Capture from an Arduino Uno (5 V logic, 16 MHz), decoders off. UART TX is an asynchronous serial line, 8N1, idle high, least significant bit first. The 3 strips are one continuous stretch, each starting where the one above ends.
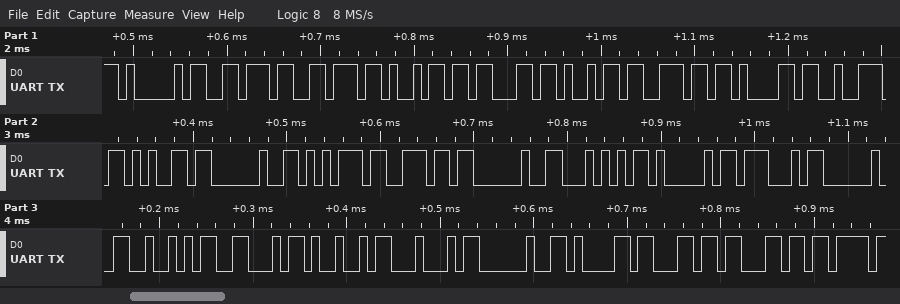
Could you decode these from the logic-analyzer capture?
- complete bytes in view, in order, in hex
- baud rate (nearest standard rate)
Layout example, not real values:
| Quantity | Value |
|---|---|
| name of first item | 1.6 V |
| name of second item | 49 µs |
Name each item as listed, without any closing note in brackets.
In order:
| Quantity | Value |
|---|---|
| complete bytes in view, in order, in hex | 0x41 0x76 0x76 0x69 0x63 0x69 0x6E 0x61 0x72 0x65 0x20 0x75 0x6E 0x20 0x54 0x41 0x47 0x20 0x52 0x46 0x49 0x44 0x20 0x61 0x6C 0x6C |
| baud rate | 115200 baud |
